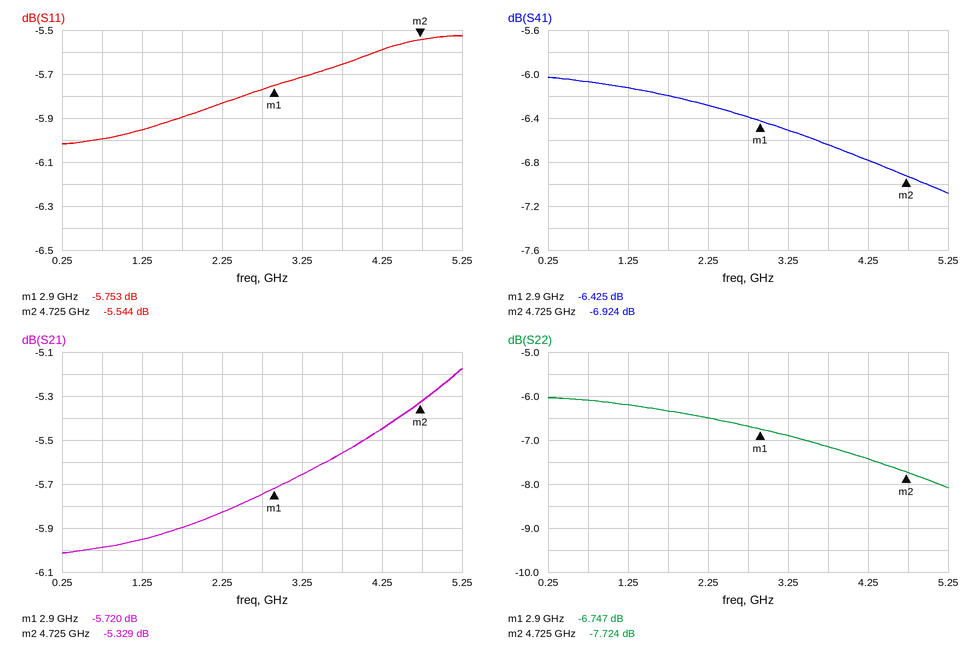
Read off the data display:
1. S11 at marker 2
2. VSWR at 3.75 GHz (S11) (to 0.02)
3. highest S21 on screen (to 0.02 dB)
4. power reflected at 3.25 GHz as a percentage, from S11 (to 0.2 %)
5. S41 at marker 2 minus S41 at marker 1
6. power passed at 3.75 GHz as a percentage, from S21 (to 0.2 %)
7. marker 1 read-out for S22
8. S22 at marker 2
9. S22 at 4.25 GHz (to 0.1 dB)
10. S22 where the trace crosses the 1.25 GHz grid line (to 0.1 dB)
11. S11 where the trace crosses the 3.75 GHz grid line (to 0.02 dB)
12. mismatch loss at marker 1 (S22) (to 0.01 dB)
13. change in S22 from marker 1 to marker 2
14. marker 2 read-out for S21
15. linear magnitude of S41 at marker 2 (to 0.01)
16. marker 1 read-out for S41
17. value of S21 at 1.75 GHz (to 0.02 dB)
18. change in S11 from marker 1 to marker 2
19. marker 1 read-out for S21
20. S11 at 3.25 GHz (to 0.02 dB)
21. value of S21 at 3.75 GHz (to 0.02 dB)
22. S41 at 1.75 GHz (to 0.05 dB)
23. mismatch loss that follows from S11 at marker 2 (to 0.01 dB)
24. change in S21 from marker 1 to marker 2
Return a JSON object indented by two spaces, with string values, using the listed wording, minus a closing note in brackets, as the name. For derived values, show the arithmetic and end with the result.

{
  "S11 at marker 2": "-5.544 dB",
  "VSWR at 3.75 GHz (S11)": "|Γ| = 10^(-5.66/20) = 0.5212; VSWR = (1 + 0.5212)/(1 − 0.5212) ≈ 3.18",
  "highest S21 on screen": "-5.18 dB",
  "power reflected at 3.25 GHz as a percentage, from S11": "10^(-5.72/10) ≈ 26.8 %",
  "S41 at marker 2 minus S41 at marker 1": "-6.924 − (-6.425) = -0.499 dB",
  "power passed at 3.75 GHz as a percentage, from S21": "10^(-5.56/10) ≈ 27.8 %",
  "marker 1 read-out for S22": "-6.747 dB",
  "S22 at marker 2": "-7.724 dB",
  "S22 at 4.25 GHz": "-7.4 dB",
  "S22 where the trace crosses the 1.25 GHz grid line": "-6.2 dB",
  "S11 where the trace crosses the 3.75 GHz grid line": "-5.66 dB",
  "mismatch loss at marker 1 (S22)": "−10 log10(1 − 10^(-6.747/10)) ≈ 1.03 dB",
  "change in S22 from marker 1 to marker 2": "-7.724 − (-6.747) = -0.977 dB",
  "marker 2 read-out for S21": "-5.329 dB",
  "linear magnitude of S41 at marker 2": "10^(-6.924/20) ≈ 0.45",
  "marker 1 read-out for S41": "-6.425 dB",
  "value of S21 at 1.75 GHz": "-5.90 dB",
  "change in S11 from marker 1 to marker 2": "-5.544 − (-5.753) = 0.209 dB",
  "marker 1 read-out for S21": "-5.720 dB",
  "S11 at 3.25 GHz": "-5.72 dB",
  "value of S21 at 3.75 GHz": "-5.56 dB",
  "S41 at 1.75 GHz": "-6.20 dB",
  "mismatch loss that follows from S11 at marker 2": "−10 log10(1 − 10^(-5.544/10)) ≈ 1.42 dB",
  "change in S21 from marker 1 to marker 2": "-5.329 − (-5.72) = 0.391 dB"
}
